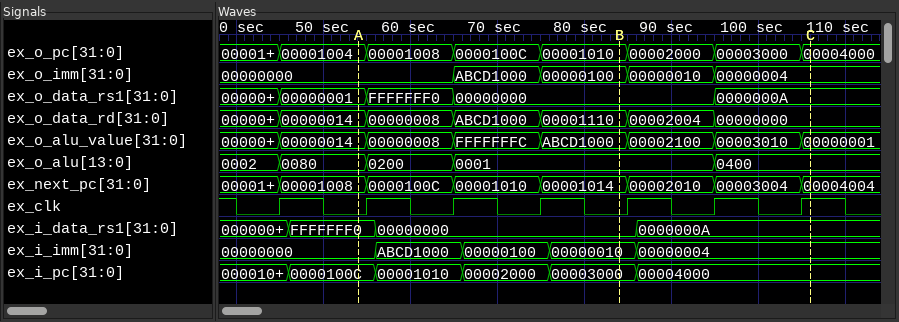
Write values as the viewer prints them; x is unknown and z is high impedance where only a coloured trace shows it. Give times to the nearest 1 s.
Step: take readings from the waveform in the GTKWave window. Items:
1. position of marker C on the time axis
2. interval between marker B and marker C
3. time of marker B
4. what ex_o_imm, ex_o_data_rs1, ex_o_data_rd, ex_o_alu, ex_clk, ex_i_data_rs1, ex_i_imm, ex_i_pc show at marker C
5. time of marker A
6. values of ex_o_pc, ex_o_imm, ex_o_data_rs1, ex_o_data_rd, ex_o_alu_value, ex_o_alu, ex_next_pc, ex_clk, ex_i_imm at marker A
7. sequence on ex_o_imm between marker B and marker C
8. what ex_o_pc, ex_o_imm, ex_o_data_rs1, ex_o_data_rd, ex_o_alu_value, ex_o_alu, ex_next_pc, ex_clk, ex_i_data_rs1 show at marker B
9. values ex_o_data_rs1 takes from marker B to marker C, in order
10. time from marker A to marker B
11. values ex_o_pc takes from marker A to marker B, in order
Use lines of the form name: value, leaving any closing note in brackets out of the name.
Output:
position of marker C on the time axis: 106 s
interval between marker B and marker C: 22 s
time of marker B: 84 s
what ex_o_imm, ex_o_data_rs1, ex_o_data_rd, ex_o_alu, ex_clk, ex_i_data_rs1, ex_i_imm, ex_i_pc show at marker C: ex_o_imm=00000004, ex_o_data_rs1=0000000A, ex_o_data_rd=00000000, ex_o_alu=0400, ex_clk=1, ex_i_data_rs1=0000000A, ex_i_imm=00000004, ex_i_pc=00004000
time of marker A: 54 s
values of ex_o_pc, ex_o_imm, ex_o_data_rs1, ex_o_data_rd, ex_o_alu_value, ex_o_alu, ex_next_pc, ex_clk, ex_i_imm at marker A: ex_o_pc=00001004, ex_o_imm=00000000, ex_o_data_rs1=00000001, ex_o_data_rd=00000014, ex_o_alu_value=00000014, ex_o_alu=0080, ex_next_pc=00001008, ex_clk=0, ex_i_imm=00000000
sequence on ex_o_imm between marker B and marker C: 00000100, 00000010, 00000004
what ex_o_pc, ex_o_imm, ex_o_data_rs1, ex_o_data_rd, ex_o_alu_value, ex_o_alu, ex_next_pc, ex_clk, ex_i_data_rs1 show at marker B: ex_o_pc=00001010, ex_o_imm=00000100, ex_o_data_rs1=00000000, ex_o_data_rd=00001110, ex_o_alu_value=ABCD1000, ex_o_alu=0001, ex_next_pc=00001014, ex_clk=0, ex_i_data_rs1=00000000
values ex_o_data_rs1 takes from marker B to marker C, in order: 00000000, 0000000A
time from marker A to marker B: 30 s
values ex_o_pc takes from marker A to marker B, in order: 00001004, 00001008, 0000100C, 00001010
